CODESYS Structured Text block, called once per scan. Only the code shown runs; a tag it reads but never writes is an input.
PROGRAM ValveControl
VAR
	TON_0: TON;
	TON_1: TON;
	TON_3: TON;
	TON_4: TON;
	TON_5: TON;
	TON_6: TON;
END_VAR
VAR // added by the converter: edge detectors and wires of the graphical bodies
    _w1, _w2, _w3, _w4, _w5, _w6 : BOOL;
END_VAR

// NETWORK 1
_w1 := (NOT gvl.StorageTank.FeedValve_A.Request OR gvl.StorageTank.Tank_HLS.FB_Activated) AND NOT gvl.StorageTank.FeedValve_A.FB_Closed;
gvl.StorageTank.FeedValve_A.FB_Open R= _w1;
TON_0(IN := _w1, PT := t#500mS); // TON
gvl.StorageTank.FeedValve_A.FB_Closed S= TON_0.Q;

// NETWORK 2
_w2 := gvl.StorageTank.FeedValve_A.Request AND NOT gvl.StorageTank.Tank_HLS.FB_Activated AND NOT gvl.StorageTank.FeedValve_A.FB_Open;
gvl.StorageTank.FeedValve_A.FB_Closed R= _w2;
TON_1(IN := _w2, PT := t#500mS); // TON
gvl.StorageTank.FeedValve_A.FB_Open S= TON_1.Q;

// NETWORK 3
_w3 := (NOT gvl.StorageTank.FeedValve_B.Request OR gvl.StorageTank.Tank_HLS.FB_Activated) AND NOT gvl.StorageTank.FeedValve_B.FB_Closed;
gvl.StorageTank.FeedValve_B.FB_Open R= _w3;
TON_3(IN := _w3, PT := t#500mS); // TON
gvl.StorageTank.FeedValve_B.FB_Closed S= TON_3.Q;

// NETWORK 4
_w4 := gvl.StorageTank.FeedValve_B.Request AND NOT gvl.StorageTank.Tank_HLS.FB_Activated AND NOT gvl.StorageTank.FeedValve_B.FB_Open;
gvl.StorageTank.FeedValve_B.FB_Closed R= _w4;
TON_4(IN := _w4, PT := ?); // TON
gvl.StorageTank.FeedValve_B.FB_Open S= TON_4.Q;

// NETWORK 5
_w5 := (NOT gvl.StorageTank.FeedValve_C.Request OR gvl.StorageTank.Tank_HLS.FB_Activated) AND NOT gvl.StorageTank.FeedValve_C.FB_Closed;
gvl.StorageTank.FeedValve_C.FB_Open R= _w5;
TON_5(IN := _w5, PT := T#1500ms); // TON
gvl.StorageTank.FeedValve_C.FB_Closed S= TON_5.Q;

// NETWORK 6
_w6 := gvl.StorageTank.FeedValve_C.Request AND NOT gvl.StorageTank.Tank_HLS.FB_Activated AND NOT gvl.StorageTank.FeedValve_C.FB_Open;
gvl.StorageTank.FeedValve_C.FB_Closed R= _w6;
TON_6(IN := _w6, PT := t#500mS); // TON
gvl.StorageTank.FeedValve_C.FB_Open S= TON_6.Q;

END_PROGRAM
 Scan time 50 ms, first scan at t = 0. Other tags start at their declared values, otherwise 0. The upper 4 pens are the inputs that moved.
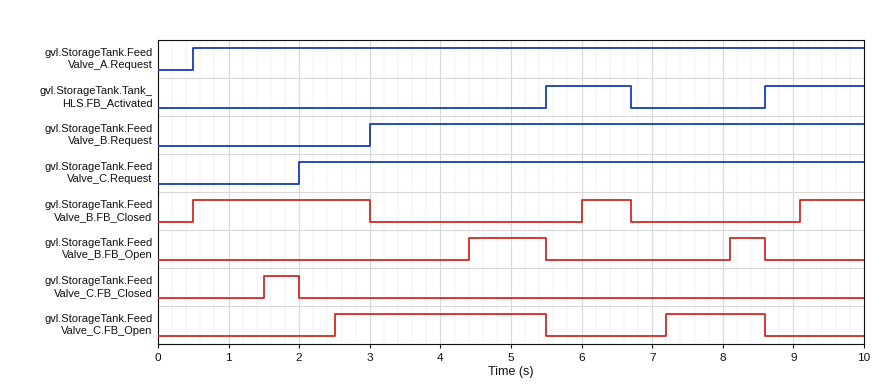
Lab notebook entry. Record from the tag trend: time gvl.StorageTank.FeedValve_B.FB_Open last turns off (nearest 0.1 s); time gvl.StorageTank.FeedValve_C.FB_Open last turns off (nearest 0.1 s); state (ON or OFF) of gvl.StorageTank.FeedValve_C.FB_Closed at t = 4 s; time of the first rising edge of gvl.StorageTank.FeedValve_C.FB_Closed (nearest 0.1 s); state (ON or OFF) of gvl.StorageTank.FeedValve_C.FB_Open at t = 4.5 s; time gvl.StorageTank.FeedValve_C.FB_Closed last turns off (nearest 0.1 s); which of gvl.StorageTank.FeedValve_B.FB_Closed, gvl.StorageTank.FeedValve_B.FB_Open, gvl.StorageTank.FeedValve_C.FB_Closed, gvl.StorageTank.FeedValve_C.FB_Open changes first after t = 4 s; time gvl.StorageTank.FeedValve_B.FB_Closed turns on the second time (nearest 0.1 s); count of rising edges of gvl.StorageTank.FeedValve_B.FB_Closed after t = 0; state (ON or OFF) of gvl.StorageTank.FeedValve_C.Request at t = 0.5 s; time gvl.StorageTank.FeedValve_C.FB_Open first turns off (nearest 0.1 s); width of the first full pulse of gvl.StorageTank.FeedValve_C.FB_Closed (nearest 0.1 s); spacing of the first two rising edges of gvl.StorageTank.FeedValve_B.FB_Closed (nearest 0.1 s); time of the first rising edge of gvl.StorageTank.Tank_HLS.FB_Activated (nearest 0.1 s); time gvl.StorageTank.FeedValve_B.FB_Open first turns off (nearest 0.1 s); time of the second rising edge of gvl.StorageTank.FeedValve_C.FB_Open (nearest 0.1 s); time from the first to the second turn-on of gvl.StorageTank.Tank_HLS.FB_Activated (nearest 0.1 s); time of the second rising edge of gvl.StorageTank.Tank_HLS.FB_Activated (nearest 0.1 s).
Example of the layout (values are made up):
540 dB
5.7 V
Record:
8.6 s
8.6 s
OFF
1.5 s
ON
2.0 s
gvl.StorageTank.FeedValve_B.FB_Open
6.0 s
3
OFF
5.5 s
0.5 s
5.5 s
5.5 s
5.5 s
7.2 s
3.1 s
8.6 s
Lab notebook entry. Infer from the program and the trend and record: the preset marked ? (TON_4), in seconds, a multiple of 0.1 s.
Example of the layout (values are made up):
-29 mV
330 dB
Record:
1.4 s
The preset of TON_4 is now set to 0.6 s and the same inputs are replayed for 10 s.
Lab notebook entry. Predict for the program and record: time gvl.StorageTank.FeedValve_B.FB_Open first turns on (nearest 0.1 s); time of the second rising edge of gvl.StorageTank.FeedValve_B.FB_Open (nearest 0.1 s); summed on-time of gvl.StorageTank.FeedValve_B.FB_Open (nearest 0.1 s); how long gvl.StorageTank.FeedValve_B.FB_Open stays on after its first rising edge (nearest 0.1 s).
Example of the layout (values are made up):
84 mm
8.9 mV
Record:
3.6 s
7.3 s
3.2 s
1.9 s
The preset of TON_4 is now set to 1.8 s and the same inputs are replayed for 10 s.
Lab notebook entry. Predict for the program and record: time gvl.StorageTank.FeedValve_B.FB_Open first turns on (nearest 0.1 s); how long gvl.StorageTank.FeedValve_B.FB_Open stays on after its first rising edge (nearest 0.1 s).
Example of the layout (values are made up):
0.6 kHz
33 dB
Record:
4.8 s
0.7 s
